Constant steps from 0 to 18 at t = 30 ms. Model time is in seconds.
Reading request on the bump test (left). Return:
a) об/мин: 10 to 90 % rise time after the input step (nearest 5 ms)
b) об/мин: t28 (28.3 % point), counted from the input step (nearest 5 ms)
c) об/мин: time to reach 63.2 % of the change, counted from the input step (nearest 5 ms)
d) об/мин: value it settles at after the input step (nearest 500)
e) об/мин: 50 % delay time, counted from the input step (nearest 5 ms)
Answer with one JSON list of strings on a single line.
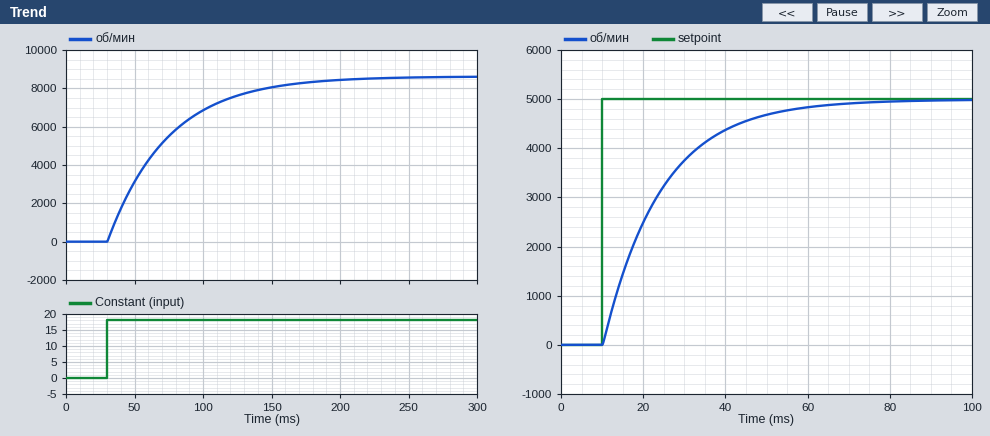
["95 ms", "15 ms", "45 ms", "8500", "30 ms"]
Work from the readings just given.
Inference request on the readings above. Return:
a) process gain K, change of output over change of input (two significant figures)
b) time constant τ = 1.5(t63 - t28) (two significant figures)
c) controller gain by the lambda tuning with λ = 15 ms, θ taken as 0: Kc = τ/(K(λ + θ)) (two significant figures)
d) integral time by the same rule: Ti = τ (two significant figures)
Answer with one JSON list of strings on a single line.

["470", "45 ms", "0.0064", "45 ms"]
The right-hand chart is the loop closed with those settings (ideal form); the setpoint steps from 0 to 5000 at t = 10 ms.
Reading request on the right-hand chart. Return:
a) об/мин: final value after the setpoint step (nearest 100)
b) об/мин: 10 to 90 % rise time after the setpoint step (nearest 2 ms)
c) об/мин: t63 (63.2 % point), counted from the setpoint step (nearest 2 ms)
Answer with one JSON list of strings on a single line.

["5000", "32 ms", "14 ms"]
